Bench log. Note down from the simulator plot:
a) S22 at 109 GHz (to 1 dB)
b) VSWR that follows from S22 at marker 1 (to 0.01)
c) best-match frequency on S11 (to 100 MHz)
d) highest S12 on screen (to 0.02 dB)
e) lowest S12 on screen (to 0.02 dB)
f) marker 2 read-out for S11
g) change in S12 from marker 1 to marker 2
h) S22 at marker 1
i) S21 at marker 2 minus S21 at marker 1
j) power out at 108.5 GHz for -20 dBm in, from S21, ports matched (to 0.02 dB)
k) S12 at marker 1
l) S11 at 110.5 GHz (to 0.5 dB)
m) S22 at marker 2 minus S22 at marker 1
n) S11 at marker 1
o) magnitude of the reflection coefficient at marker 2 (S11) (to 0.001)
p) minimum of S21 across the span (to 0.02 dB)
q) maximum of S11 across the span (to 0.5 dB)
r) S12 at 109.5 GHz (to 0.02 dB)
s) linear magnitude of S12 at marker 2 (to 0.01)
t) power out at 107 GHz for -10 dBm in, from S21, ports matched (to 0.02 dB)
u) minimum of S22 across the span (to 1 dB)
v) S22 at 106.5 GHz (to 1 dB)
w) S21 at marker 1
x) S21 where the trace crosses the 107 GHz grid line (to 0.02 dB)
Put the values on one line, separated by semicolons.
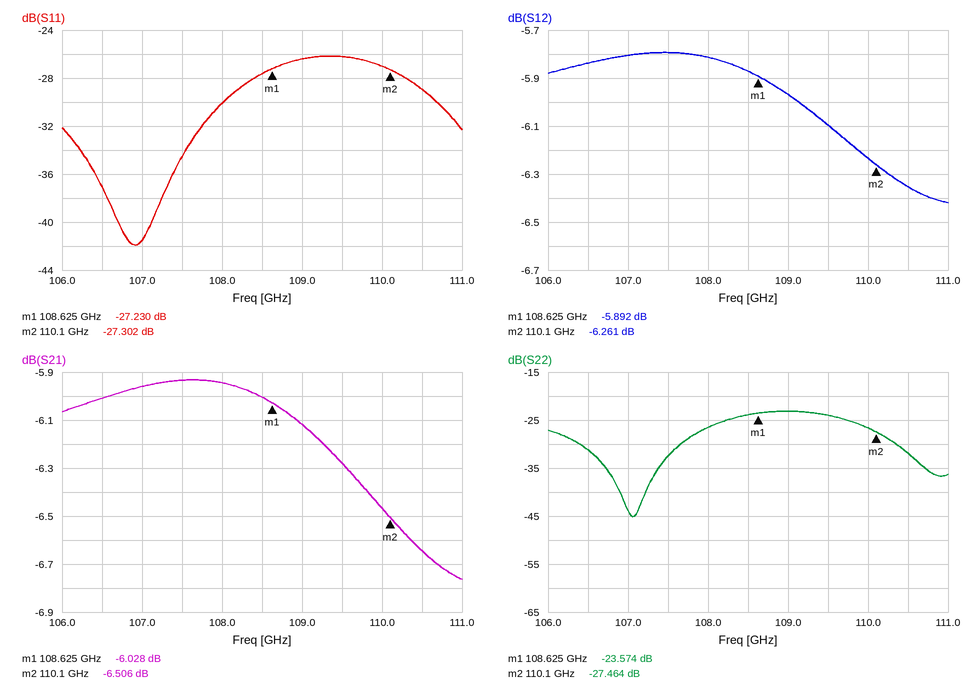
-23 dB; 1.14; 106.9 GHz; -5.80 dB; -6.42 dB; -27.302 dB; -0.369 dB; -23.574 dB; -0.478 dB; -26.00 dBm; -5.892 dB; -29.0 dB; -3.890 dB; -27.230 dB; 0.043; -6.76 dB; -26.0 dB; -6.10 dB; 0.49; -15.96 dBm; -45 dB; -31 dB; -6.028 dB; -5.96 dB
